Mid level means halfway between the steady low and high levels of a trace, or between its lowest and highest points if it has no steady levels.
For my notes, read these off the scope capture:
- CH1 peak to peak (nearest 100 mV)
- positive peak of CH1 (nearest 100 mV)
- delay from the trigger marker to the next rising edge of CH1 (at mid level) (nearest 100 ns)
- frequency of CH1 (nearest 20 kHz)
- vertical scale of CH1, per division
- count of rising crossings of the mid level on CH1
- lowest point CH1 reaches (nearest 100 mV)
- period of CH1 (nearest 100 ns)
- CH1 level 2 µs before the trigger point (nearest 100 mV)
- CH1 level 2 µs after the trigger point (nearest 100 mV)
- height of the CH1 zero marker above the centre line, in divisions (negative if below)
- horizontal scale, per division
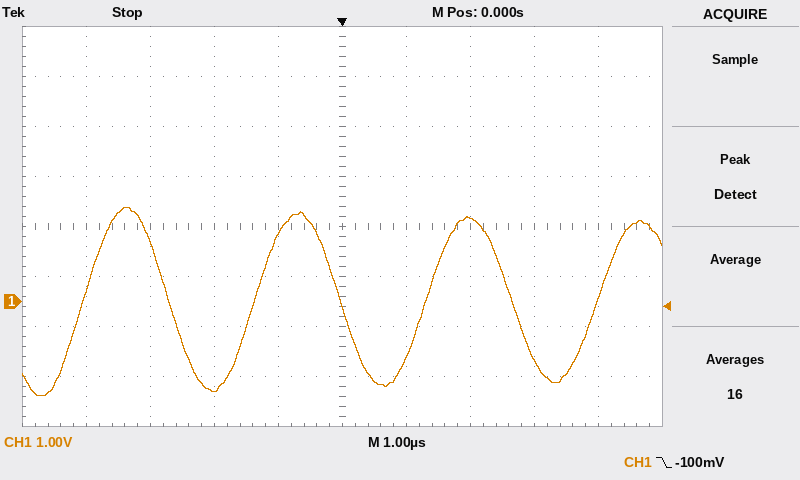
3.8 V
1.9 V
1.3 µs
380 kHz
1 V
4
-1.9 V
2.7 µs
-1.8 V
1.7 V
-1.5 div
1 µs
